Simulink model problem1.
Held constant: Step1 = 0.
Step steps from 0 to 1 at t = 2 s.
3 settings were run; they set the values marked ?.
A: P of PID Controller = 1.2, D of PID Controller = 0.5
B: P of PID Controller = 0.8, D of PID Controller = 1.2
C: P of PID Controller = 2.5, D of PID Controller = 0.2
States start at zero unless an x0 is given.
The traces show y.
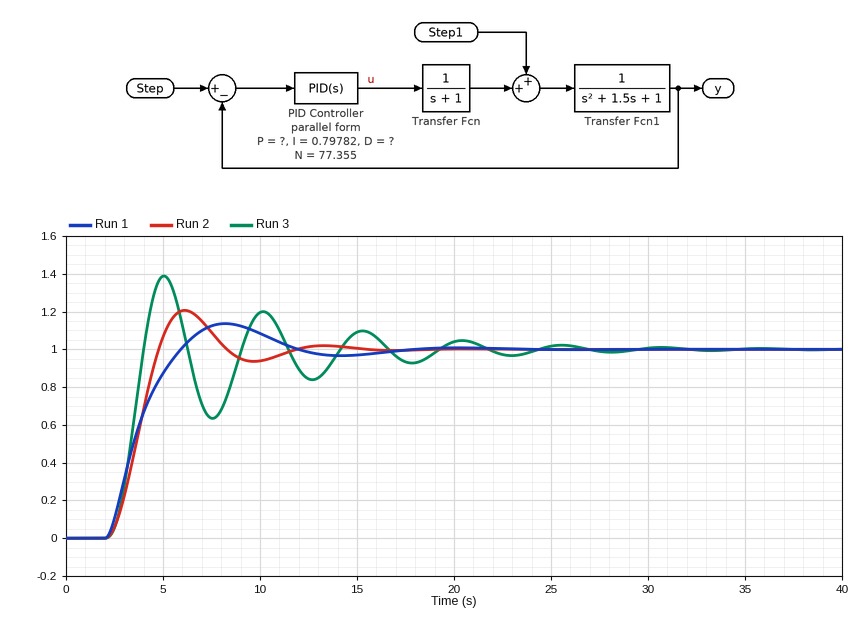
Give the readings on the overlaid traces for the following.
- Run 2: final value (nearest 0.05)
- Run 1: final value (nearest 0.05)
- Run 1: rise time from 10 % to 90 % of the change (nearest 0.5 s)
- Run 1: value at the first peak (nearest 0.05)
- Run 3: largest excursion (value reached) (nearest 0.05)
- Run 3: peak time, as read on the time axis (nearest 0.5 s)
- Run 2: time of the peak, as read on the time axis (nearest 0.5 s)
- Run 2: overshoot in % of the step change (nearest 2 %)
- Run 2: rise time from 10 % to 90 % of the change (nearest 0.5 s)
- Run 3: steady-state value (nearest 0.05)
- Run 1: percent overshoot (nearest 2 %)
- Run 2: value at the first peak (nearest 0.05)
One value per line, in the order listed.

1.00
1.00
2.5 s
1.15
1.40
5.0 s
6.0 s
20 %
2.0 s
1.00
14 %
1.20
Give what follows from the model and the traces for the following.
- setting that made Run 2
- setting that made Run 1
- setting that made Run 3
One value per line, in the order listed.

A
B
C
